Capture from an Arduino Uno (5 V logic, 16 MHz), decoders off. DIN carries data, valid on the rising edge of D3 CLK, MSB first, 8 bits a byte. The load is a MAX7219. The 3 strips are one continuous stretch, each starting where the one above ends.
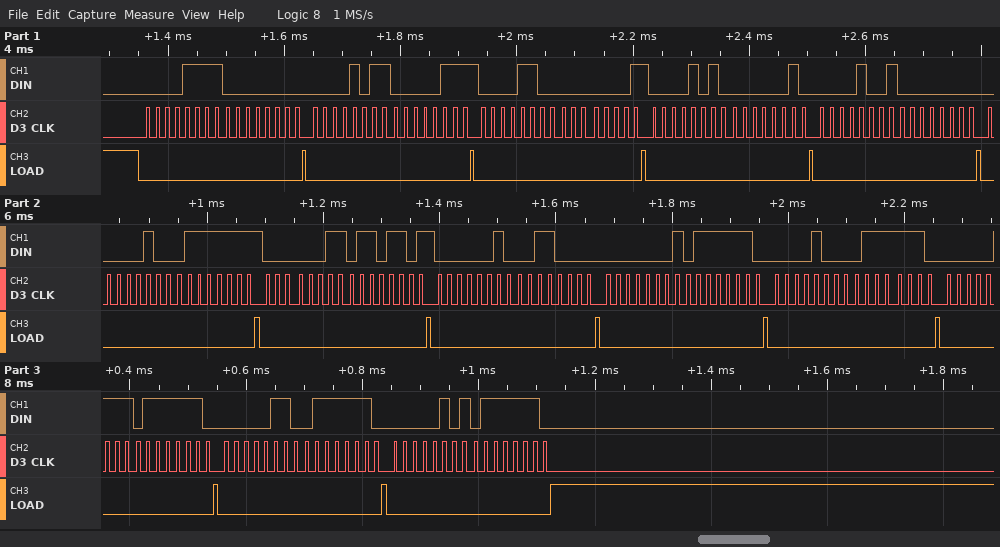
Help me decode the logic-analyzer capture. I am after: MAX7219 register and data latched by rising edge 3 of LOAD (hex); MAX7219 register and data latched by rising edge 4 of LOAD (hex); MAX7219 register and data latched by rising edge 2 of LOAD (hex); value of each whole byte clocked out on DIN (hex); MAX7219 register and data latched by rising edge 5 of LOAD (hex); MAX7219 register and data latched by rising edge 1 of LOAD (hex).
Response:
register 0xC, data 0x01
register 0xA, data 0x02
register 0xB, data 0x07
0F 00 0B 07 0C 01 0A 02 09 00 04 7F 03 6D 02 30 01 7E 08 7E 07 7E 06 7E 05 7E
register 0x9, data 0x00
register 0xF, data 0x00
